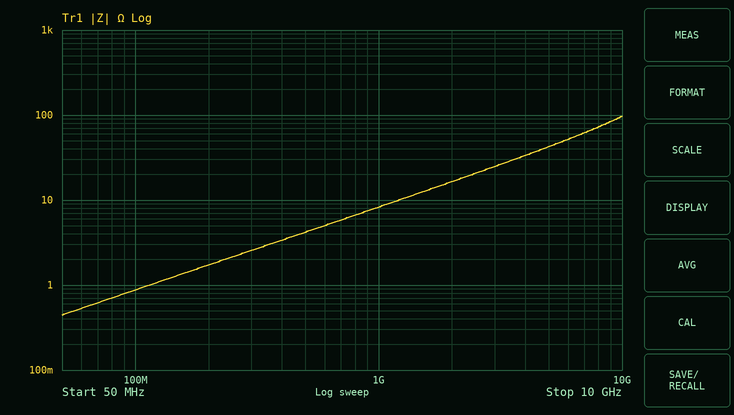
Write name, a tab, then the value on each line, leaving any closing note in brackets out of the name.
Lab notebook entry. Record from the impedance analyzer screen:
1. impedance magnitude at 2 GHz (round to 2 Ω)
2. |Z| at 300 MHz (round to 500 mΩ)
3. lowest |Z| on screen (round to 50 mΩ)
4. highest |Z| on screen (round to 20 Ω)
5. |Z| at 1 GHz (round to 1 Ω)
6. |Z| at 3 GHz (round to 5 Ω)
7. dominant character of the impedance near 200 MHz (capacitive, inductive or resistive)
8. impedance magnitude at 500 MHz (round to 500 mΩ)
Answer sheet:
impedance magnitude at 2 GHz	16 Ω
|Z| at 300 MHz	2.5 Ω
lowest |Z| on screen	450 mΩ
highest |Z| on screen	100 Ω
|Z| at 1 GHz	8 Ω
|Z| at 3 GHz	25 Ω
dominant character of the impedance near 200 MHz	inductive
impedance magnitude at 500 MHz	4.0 Ω
